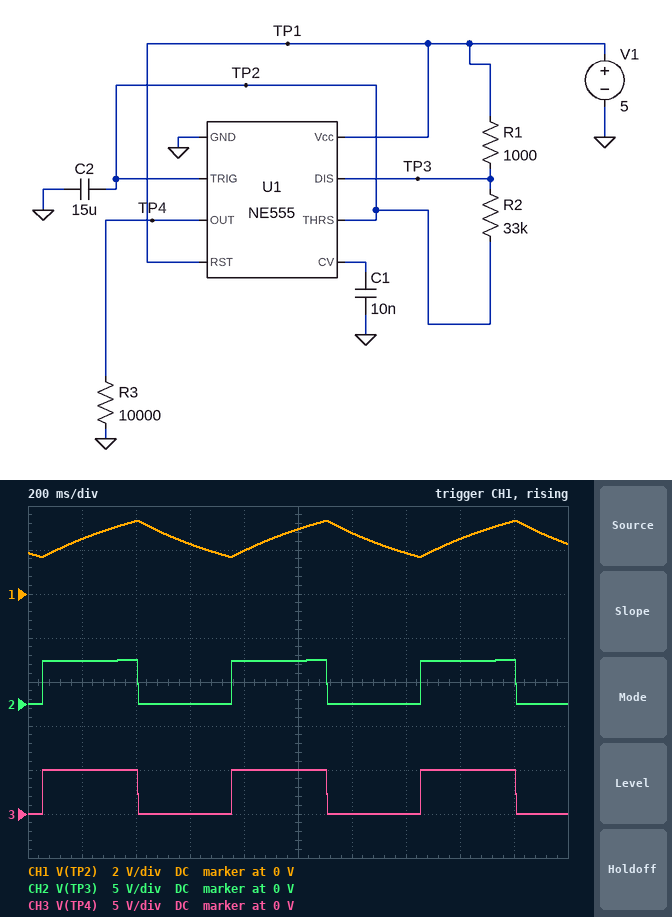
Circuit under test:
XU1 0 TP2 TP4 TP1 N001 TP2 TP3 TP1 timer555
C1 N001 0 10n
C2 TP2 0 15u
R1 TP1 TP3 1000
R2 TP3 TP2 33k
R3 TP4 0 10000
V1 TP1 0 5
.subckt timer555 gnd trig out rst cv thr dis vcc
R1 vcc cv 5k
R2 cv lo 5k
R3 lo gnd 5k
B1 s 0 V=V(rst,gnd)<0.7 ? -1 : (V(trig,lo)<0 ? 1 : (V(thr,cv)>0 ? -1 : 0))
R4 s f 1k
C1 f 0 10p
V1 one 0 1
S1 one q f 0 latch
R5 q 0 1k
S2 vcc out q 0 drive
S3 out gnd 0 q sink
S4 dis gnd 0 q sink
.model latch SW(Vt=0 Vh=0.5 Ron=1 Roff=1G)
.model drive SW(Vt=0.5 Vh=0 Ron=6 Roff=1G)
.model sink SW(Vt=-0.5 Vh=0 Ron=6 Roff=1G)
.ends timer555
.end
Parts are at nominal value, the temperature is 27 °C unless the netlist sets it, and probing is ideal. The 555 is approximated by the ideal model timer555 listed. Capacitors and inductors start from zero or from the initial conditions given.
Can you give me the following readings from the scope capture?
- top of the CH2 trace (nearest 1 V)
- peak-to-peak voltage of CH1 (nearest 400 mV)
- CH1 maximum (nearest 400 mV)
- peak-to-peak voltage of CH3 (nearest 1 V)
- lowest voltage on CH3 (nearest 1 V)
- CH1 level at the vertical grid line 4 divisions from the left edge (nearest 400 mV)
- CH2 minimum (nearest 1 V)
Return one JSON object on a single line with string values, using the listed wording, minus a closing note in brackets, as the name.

{"top of the CH2 trace": "5 V", "peak-to-peak voltage of CH1": "1.6 V", "CH1 maximum": "3.2 V", "peak-to-peak voltage of CH3": "5 V", "lowest voltage on CH3": "0 V", "CH1 level at the vertical grid line 4 divisions from the left edge": "2.0 V", "CH2 minimum": "0 V"}
